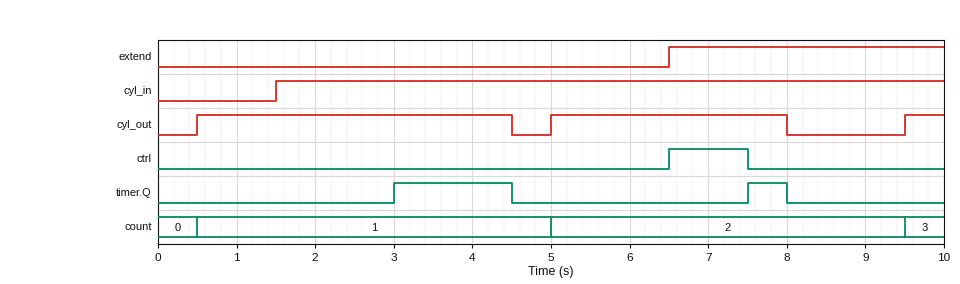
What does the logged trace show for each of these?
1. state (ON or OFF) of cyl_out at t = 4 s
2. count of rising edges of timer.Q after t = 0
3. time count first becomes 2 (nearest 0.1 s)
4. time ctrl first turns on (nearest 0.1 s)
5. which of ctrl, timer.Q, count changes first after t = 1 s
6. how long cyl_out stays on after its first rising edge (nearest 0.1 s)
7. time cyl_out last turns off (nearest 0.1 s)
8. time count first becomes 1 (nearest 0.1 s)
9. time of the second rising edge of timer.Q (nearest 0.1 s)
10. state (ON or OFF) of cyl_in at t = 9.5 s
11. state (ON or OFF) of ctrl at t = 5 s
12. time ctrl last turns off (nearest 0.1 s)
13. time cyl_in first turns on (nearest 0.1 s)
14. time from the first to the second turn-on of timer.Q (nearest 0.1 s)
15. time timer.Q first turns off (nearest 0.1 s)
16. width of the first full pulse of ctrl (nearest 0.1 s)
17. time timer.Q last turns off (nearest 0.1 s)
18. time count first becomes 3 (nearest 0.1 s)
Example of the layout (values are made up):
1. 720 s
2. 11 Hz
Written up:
1. ON
2. 2
3. 5.0 s
4. 6.5 s
5. timer.Q
6. 4.0 s
7. 8.0 s
8. 0.5 s
9. 7.5 s
10. ON
11. OFF
12. 7.5 s
13. 1.5 s
14. 4.5 s
15. 4.5 s
16. 1.0 s
17. 8.0 s
18. 9.5 s
